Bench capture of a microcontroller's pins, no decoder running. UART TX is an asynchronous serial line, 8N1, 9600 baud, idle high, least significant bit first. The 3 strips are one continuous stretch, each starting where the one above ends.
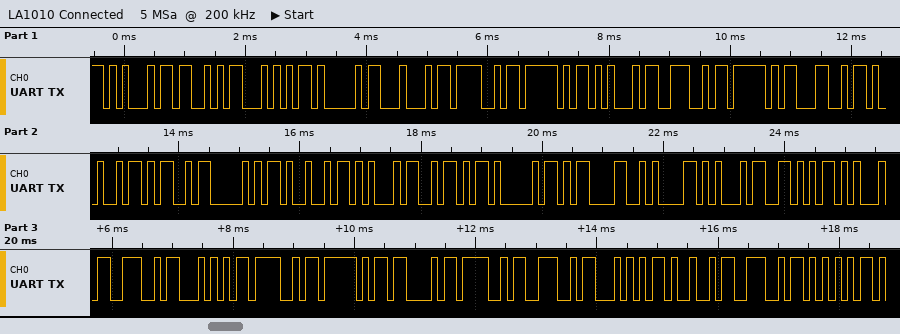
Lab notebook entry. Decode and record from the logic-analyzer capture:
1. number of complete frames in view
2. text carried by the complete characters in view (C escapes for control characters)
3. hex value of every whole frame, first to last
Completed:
34
"ESTADO_EN_LIMPIEZA\r\nEVENTO_CONTINU"
45 53 54 41 44 4F 5F 45 4E 5F 4C 49 4D 50 49 45 5A 41 0D 0A 45 56 45 4E 54 4F 5F 43 4F 4E 54 49 4E 55
